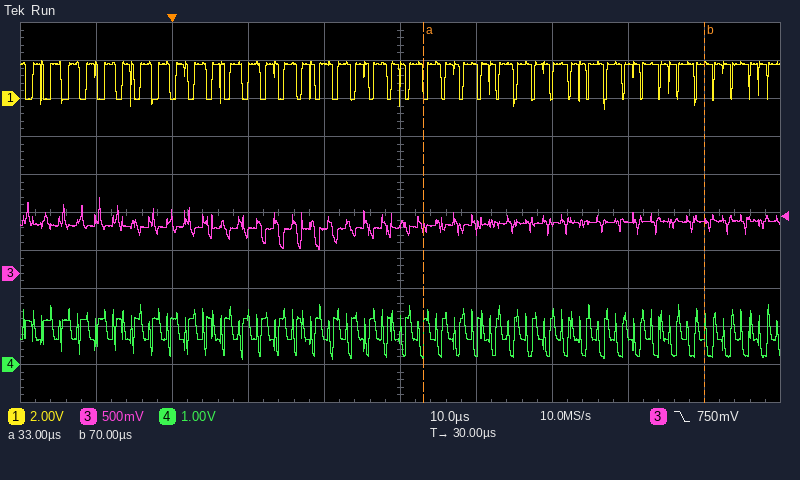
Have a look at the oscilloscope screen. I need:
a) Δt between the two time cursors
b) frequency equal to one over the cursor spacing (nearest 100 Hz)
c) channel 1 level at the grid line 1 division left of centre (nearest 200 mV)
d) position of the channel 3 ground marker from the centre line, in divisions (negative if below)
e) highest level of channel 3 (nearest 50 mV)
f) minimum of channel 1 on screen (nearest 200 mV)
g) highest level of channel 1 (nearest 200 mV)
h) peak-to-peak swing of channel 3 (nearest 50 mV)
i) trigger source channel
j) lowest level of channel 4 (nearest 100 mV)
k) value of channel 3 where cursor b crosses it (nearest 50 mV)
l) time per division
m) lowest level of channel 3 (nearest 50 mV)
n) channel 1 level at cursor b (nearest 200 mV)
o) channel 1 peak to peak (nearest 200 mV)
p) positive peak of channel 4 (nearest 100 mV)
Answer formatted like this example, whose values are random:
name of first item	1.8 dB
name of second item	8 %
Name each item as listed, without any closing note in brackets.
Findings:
Δt between the two time cursors	37 µs
frequency equal to one over the cursor spacing	27.0 kHz
channel 1 level at the grid line 1 division left of centre	1.8 V
position of the channel 3 ground marker from the centre line, in divisions	-1.6 div
highest level of channel 3	1.00 V
minimum of channel 1 on screen	-600 mV
highest level of channel 1	2.0 V
peak-to-peak swing of channel 3	700 mV
trigger source channel	channel 3
lowest level of channel 4	100 mV
value of channel 3 where cursor b crosses it	700 mV
time per division	10 µs
lowest level of channel 3	300 mV
channel 1 level at cursor b	1.8 V
channel 1 peak to peak	2.6 V
positive peak of channel 4	1.6 V
